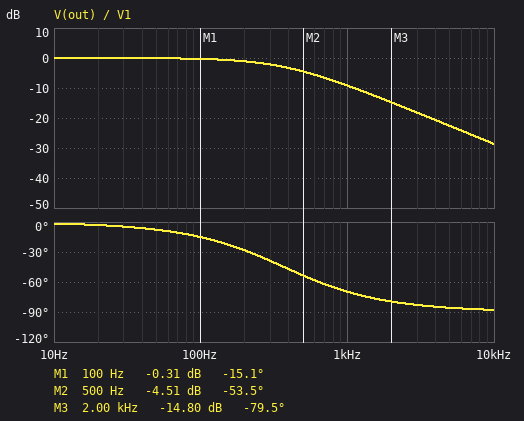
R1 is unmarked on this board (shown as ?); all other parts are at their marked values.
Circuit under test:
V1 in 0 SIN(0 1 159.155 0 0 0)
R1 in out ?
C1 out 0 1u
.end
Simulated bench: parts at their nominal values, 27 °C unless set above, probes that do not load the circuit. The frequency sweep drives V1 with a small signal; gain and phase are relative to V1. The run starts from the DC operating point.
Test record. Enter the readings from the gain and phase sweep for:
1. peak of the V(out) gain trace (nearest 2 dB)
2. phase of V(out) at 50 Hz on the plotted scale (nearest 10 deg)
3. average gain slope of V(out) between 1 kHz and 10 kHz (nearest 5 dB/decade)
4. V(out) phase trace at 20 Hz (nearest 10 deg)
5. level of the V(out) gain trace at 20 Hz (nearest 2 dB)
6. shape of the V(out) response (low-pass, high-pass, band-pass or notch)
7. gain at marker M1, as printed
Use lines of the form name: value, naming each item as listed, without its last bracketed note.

peak of the V(out) gain trace: 0 dB
phase of V(out) at 50 Hz on the plotted scale: -10 deg
average gain slope of V(out) between 1 kHz and 10 kHz: -20 dB/decade
V(out) phase trace at 20 Hz: 0 deg
level of the V(out) gain trace at 20 Hz: 0 dB
shape of the V(out) response: low-pass
gain at marker M1, as printed: -0.31 dB
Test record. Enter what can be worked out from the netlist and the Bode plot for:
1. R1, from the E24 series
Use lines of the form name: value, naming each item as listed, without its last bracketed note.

R1, from the E24 series: 430 Ω
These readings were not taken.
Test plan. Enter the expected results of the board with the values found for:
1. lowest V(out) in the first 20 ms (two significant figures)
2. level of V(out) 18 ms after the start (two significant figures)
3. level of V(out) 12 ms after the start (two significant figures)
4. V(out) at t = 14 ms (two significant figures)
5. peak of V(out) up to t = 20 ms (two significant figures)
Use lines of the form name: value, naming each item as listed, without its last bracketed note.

lowest V(out) in the first 20 ms: -920 mV
level of V(out) 18 ms after the start: -870 mV
level of V(out) 12 ms after the start: -760 mV
V(out) at t = 14 ms: 790 mV
peak of V(out) up to t = 20 ms: 920 mV
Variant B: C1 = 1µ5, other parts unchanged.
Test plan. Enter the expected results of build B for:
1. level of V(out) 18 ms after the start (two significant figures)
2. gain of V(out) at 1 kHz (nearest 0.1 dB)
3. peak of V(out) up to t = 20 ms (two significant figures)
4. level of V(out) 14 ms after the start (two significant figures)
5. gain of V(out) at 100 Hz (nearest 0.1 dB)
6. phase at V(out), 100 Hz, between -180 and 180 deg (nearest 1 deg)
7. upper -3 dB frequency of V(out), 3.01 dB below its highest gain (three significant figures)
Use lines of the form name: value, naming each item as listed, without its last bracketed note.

level of V(out) 18 ms after the start: -830 mV
gain of V(out) at 1 kHz: -12.4 dB
peak of V(out) up to t = 20 ms: 860 mV
level of V(out) 14 ms after the start: 640 mV
gain of V(out) at 100 Hz: -0.7 dB
phase at V(out), 100 Hz, between -180 and 180 deg: -22 deg
upper -3 dB frequency of V(out), 3.01 dB below its highest gain: 247 Hz
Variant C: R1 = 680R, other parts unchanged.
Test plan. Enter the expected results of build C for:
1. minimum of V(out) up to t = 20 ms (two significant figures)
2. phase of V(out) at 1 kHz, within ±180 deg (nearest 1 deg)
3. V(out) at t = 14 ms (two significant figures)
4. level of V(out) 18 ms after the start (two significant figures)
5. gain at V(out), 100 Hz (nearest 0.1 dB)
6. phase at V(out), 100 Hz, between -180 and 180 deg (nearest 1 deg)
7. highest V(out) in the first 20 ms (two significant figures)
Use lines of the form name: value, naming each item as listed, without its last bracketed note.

minimum of V(out) up to t = 20 ms: -830 mV
phase of V(out) at 1 kHz, within ±180 deg: -77 deg
V(out) at t = 14 ms: 610 mV
level of V(out) 18 ms after the start: -820 mV
gain at V(out), 100 Hz: -0.7 dB
phase at V(out), 100 Hz, between -180 and 180 deg: -23 deg
highest V(out) in the first 20 ms: 850 mV
